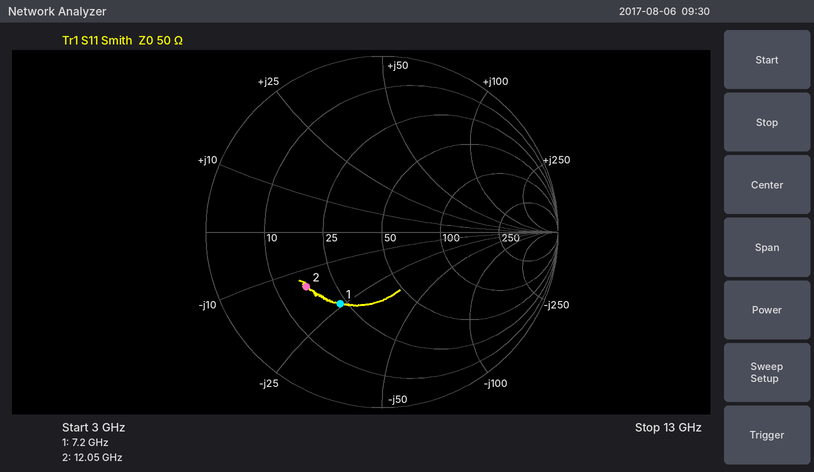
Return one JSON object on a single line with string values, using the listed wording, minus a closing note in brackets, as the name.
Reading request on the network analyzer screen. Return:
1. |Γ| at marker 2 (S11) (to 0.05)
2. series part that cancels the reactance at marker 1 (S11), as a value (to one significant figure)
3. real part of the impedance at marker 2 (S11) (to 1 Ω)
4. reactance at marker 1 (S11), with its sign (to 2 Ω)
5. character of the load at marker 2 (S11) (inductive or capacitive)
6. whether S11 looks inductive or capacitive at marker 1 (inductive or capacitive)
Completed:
{"|Γ| at marker 2 (S11)": "0.55", "series part that cancels the reactance at marker 1 (S11), as a value": "500 pH", "real part of the impedance at marker 2 (S11)": "17 Ω", "reactance at marker 1 (S11), with its sign": "-24 Ω", "character of the load at marker 2 (S11)": "capacitive", "whether S11 looks inductive or capacitive at marker 1": "capacitive"}
